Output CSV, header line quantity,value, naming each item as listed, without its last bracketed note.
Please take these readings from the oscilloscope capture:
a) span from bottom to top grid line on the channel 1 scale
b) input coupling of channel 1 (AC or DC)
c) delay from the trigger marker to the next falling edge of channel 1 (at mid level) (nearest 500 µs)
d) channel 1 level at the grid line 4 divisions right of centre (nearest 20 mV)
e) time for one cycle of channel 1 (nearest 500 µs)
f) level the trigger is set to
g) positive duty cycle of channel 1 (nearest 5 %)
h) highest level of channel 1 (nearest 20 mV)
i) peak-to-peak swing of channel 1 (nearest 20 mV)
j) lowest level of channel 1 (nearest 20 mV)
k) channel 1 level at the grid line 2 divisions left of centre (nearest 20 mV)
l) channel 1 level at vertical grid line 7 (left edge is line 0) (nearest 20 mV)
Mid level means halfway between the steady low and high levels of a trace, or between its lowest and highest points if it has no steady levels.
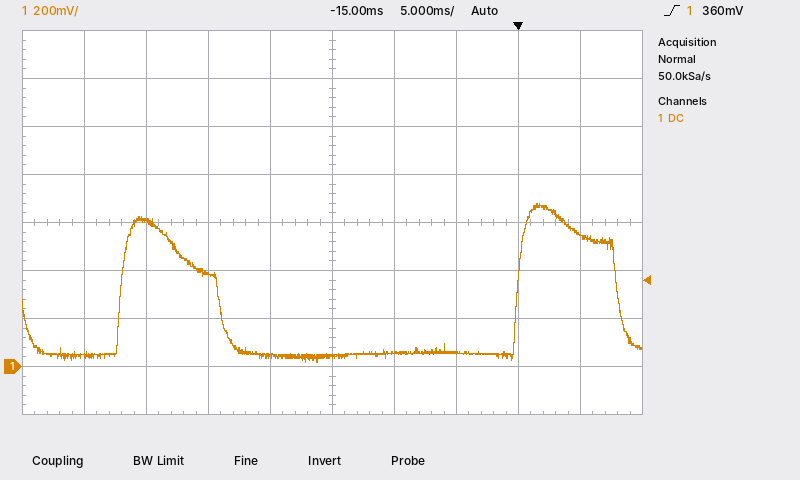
quantity,value
span from bottom to top grid line on the channel 1 scale,1.6 V
input coupling of channel 1,DC
delay from the trigger marker to the next falling edge of channel 1 (at mid level),8.0 ms
channel 1 level at the grid line 4 divisions right of centre,540 mV
time for one cycle of channel 1,32.0 ms
level the trigger is set to,360 mV
positive duty cycle of channel 1,25 %
highest level of channel 1,680 mV
peak-to-peak swing of channel 1,660 mV
lowest level of channel 1,20 mV
channel 1 level at the grid line 2 divisions left of centre,380 mV
channel 1 level at vertical grid line 7 (left edge is line 0),60 mV
